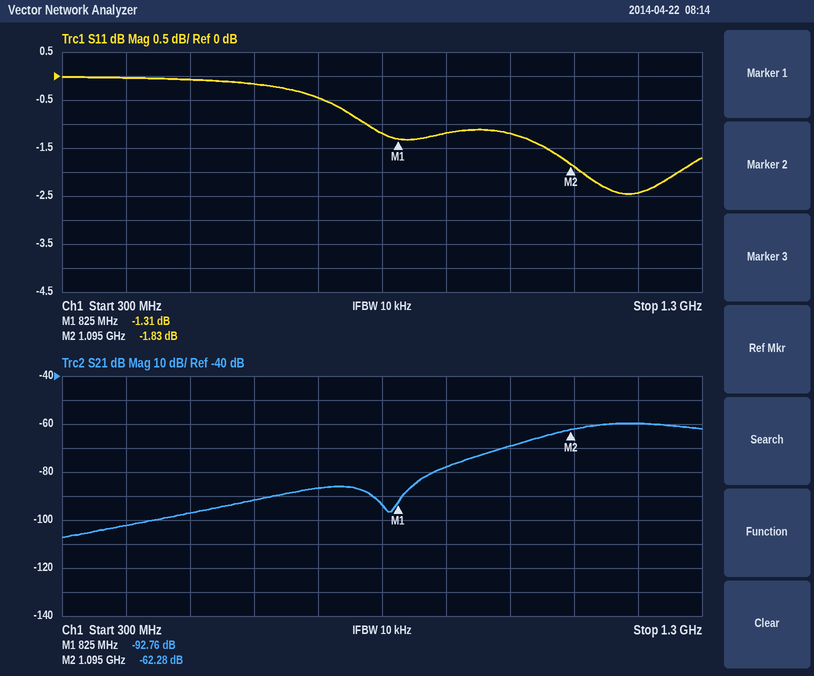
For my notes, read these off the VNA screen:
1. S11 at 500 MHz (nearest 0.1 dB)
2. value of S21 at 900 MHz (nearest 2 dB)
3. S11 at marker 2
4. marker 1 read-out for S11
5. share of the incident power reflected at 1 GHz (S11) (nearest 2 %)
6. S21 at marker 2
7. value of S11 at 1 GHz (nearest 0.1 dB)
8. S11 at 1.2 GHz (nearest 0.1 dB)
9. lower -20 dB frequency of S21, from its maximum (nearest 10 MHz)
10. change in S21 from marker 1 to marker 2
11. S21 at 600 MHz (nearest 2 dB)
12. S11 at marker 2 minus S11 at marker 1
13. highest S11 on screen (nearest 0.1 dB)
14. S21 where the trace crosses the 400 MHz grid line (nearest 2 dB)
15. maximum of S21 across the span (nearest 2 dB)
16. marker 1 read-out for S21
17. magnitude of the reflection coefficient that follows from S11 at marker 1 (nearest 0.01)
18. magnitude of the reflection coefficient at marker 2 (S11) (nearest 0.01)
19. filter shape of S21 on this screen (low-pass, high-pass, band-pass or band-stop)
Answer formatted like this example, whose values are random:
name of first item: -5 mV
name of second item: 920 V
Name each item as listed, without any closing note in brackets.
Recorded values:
S11 at 500 MHz: -0.1 dB
value of S21 at 900 MHz: -78 dB
S11 at marker 2: -1.83 dB
marker 1 read-out for S11: -1.31 dB
share of the incident power reflected at 1 GHz (S11): 76 %
S21 at marker 2: -62.28 dB
value of S11 at 1 GHz: -1.2 dB
S11 at 1.2 GHz: -2.4 dB
lower -20 dB frequency of S21, from its maximum: 880 MHz
change in S21 from marker 1 to marker 2: 30.48 dB
S21 at 600 MHz: -92 dB
S11 at marker 2 minus S11 at marker 1: -0.52 dB
highest S11 on screen: 0.0 dB
S21 where the trace crosses the 400 MHz grid line: -102 dB
maximum of S21 across the span: -60 dB
marker 1 read-out for S21: -92.76 dB
magnitude of the reflection coefficient that follows from S11 at marker 1: 0.86
magnitude of the reflection coefficient at marker 2 (S11): 0.81
filter shape of S21 on this screen: high-pass
